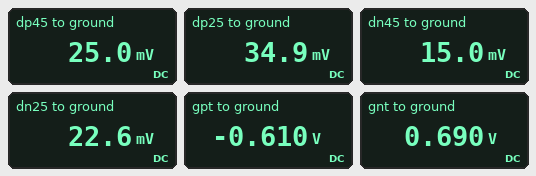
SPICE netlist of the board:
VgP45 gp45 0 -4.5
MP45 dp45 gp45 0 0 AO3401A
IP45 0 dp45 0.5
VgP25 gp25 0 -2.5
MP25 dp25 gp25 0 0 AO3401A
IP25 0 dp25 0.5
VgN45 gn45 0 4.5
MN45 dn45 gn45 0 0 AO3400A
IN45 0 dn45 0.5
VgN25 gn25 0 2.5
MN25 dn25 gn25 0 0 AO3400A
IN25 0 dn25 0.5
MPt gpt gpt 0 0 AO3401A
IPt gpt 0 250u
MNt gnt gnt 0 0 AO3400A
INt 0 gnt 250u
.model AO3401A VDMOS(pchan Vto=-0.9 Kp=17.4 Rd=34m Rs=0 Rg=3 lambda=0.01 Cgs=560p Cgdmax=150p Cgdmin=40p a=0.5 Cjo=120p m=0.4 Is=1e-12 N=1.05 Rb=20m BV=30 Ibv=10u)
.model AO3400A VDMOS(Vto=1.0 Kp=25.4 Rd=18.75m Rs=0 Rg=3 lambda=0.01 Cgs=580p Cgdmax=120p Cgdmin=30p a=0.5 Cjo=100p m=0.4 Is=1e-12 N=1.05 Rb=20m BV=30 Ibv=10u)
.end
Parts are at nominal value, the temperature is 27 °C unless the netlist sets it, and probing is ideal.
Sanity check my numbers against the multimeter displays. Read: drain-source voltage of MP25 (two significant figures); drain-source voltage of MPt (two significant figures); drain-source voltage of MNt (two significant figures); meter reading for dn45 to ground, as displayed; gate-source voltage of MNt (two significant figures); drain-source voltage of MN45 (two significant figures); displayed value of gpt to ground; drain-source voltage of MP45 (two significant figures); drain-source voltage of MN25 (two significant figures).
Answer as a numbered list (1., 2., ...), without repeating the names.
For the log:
1. 35 mV
2. -610 mV
3. 690 mV
4. 15.0 mV
5. 690 mV
6. 15 mV
7. -0.610 V
8. 25 mV
9. 23 mV
